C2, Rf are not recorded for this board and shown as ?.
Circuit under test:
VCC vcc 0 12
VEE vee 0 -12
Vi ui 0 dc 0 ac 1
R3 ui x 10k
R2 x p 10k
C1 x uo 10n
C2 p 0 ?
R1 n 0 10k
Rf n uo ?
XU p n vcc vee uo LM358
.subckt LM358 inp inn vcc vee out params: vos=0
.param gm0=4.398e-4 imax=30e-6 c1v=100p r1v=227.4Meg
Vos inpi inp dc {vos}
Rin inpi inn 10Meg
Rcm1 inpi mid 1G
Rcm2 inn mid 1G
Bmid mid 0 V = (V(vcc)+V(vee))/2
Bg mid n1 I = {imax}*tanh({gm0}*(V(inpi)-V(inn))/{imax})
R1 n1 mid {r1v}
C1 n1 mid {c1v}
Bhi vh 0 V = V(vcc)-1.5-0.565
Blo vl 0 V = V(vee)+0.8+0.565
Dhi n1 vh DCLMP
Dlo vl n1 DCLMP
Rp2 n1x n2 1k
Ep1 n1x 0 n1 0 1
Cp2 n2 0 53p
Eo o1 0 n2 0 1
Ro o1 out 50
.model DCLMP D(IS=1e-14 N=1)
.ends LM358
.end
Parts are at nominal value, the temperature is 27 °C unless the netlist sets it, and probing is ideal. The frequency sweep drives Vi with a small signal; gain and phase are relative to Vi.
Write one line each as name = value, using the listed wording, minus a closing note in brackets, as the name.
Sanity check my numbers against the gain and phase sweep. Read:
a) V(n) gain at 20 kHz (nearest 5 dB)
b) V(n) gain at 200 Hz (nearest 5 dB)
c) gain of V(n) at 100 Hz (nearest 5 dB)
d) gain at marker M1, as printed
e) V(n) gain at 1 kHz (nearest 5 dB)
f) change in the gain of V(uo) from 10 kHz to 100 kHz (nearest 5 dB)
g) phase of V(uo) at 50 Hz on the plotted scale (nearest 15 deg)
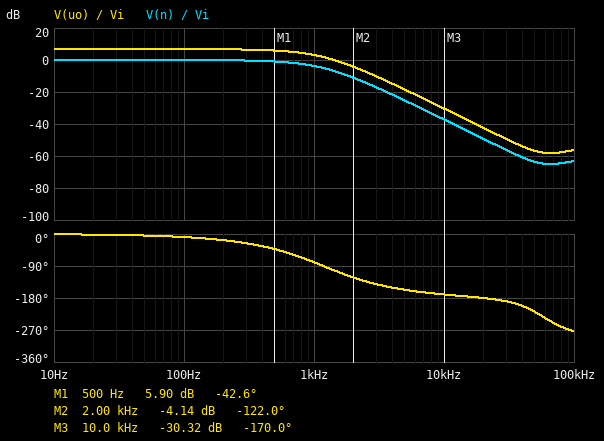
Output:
V(n) gain at 20 kHz = -50 dB
V(n) gain at 200 Hz = 0 dB
gain of V(n) at 100 Hz = 0 dB
gain at marker M1, as printed = 5.90 dB
V(n) gain at 1 kHz = -5 dB
change in the gain of V(uo) from 10 kHz to 100 kHz = -25 dB
phase of V(uo) at 50 Hz on the plotted scale = 0 deg
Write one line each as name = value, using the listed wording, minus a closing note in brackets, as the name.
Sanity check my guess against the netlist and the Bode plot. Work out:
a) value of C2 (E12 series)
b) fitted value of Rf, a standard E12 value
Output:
value of C2 = 18 nF
fitted value of Rf, a standard E12 value = 12 kΩ
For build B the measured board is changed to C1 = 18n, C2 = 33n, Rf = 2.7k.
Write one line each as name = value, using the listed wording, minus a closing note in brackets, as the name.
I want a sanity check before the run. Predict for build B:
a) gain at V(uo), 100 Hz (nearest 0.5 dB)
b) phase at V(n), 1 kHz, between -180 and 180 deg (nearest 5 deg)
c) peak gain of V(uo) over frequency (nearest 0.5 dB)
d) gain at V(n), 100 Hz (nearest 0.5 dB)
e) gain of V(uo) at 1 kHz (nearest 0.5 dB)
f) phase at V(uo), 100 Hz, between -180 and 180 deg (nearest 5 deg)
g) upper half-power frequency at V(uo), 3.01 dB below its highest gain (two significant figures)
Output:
gain at V(uo), 100 Hz = 1.5 dB
phase at V(n), 1 kHz, between -180 and 180 deg = -110 deg
peak gain of V(uo) over frequency = 2.0 dB
gain at V(n), 100 Hz = -0.5 dB
gain of V(uo) at 1 kHz = -10.0 dB
phase at V(uo), 100 Hz, between -180 and 180 deg = -20 deg
upper half-power frequency at V(uo), 3.01 dB below its highest gain = 310 Hz
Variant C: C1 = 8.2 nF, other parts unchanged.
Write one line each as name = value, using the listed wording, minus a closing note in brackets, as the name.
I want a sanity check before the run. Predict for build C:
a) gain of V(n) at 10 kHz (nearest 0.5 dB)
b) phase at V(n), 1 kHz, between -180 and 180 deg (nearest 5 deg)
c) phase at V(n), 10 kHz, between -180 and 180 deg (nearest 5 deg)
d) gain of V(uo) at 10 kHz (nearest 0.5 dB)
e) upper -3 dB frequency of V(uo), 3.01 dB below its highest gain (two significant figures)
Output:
gain of V(n) at 10 kHz = -35.5 dB
phase at V(n), 1 kHz, between -180 and 180 deg = -75 deg
phase at V(n), 10 kHz, between -180 and 180 deg = -165 deg
gain of V(uo) at 10 kHz = -28.5 dB
upper -3 dB frequency of V(uo), 3.01 dB below its highest gain = 760 Hz
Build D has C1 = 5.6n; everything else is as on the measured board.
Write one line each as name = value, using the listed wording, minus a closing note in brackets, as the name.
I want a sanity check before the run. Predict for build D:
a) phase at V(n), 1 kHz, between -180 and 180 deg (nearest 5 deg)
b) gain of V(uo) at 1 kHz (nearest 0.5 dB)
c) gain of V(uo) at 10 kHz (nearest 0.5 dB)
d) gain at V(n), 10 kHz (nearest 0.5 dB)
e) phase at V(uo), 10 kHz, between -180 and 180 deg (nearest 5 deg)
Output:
phase at V(n), 1 kHz, between -180 and 180 deg = -70 deg
gain of V(uo) at 1 kHz = 1.0 dB
gain of V(uo) at 10 kHz = -26.0 dB
gain at V(n), 10 kHz = -32.5 dB
phase at V(uo), 10 kHz, between -180 and 180 deg = -155 deg
